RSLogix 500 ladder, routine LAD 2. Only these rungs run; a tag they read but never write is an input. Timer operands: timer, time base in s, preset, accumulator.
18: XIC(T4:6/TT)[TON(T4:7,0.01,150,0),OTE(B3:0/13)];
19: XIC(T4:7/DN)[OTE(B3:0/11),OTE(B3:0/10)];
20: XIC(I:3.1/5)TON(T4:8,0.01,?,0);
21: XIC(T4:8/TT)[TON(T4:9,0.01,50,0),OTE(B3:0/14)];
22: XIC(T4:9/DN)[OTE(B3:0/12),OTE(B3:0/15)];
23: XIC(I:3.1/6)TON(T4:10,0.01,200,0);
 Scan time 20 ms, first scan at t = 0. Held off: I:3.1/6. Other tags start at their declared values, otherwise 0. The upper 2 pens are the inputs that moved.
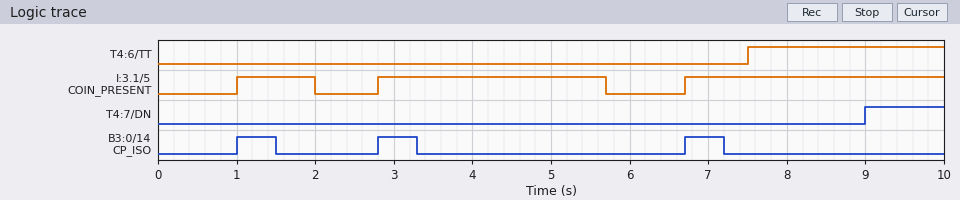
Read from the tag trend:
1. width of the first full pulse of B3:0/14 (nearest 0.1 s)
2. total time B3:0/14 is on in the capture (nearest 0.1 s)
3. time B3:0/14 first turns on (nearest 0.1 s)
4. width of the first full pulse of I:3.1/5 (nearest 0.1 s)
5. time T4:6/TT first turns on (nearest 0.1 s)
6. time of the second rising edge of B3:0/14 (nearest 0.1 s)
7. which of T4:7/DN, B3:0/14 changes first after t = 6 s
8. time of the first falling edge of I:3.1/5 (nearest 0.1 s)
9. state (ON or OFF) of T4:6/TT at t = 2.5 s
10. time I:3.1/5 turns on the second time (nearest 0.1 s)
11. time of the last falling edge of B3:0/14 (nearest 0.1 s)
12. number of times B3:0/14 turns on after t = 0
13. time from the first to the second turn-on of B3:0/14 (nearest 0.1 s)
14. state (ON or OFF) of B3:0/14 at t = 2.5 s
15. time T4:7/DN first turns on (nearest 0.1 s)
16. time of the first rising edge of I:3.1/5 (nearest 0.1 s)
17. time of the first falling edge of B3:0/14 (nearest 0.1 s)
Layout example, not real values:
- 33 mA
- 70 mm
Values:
- 0.5 s
- 1.5 s
- 1.0 s
- 1.0 s
- 7.5 s
- 2.8 s
- B3:0/14
- 2.0 s
- OFF
- 2.8 s
- 7.2 s
- 3
- 1.8 s
- OFF
- 9.0 s
- 1.0 s
- 1.5 s
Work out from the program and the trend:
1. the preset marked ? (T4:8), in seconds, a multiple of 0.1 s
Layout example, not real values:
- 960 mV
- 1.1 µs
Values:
- 0.5 s
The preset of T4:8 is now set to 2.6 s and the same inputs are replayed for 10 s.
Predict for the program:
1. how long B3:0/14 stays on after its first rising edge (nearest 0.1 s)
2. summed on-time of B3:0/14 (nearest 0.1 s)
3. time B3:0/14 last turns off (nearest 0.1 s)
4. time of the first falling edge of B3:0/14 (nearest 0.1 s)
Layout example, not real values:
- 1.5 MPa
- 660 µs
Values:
- 1.0 s
- 6.2 s
- 9.3 s
- 2.0 s
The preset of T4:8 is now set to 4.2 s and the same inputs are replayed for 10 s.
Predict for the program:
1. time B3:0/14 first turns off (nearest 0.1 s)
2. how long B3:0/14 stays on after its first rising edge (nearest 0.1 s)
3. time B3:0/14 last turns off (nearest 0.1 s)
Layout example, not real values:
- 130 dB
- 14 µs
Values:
- 2.0 s
- 1.0 s
- 5.7 s
